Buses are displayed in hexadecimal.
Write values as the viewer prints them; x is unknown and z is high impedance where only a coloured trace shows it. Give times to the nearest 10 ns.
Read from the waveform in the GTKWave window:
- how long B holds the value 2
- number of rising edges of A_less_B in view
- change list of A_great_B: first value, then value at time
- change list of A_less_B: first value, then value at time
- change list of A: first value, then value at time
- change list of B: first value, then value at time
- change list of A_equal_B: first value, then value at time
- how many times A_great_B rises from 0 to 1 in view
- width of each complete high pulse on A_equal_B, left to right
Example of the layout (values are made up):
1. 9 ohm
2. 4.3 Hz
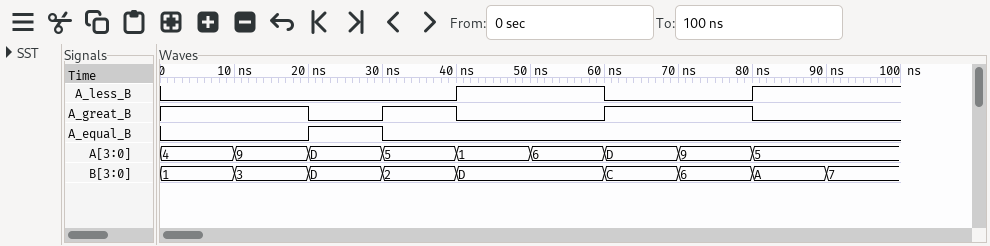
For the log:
1. 10 ns
2. 2
3. 1, 0 at 20 ns, 1 at 30 ns, 0 at 40 ns, 1 at 60 ns, 0 at 80 ns
4. 0, 1 at 40 ns, 0 at 60 ns, 1 at 80 ns
5. 4, 9 at 10 ns, D at 20 ns, 5 at 30 ns, 1 at 40 ns, 6 at 50 ns, D at 60 ns, 9 at 70 ns, 5 at 80 ns
6. 1, 3 at 10 ns, D at 20 ns, 2 at 30 ns, D at 40 ns, C at 60 ns, 6 at 70 ns, A at 80 ns, 7 at 90 ns
7. 0, 1 at 20 ns, 0 at 30 ns
8. 2
9. 10 ns
